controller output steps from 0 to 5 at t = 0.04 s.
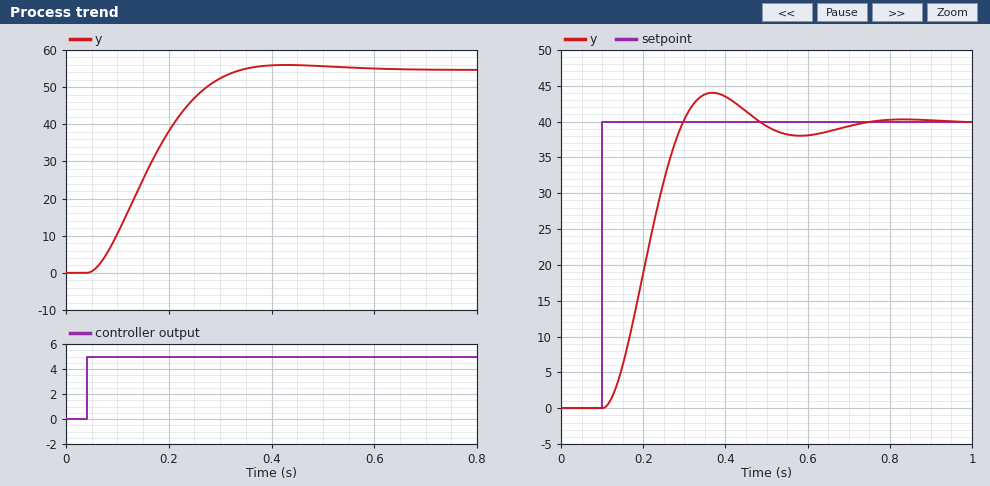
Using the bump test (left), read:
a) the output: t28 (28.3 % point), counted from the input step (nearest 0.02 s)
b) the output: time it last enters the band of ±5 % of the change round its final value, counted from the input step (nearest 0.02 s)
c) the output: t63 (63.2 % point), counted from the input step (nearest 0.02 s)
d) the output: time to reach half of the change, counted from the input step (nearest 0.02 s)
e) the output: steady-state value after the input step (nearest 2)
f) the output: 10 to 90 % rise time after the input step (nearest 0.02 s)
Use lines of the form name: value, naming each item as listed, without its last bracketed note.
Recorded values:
the output: t28 (28.3 % point), counted from the input step: 0.08 s
the output: time it last enters the band of ±5 % of the change round its final value, counted from the input step: 0.26 s
the output: t63 (63.2 % point), counted from the input step: 0.14 s
the output: time to reach half of the change, counted from the input step: 0.12 s
the output: steady-state value after the input step: 54
the output: 10 to 90 % rise time after the input step: 0.18 s
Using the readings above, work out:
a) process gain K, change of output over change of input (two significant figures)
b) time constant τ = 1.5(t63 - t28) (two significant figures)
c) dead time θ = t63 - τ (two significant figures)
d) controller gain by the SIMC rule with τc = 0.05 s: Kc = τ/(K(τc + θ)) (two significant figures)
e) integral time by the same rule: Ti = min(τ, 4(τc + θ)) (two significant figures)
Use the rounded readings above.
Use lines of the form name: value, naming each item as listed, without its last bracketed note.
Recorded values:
process gain K, change of output over change of input: 11
time constant τ = 1.5(t63 - t28): 0.090 s
dead time θ = t63 - τ: 0.050 s
controller gain by the SIMC rule with τc = 0.05 s: Kc = τ/(K(τc + θ)): 0.082
integral time by the same rule: Ti = min(τ, 4(τc + θ)): 0.090 s
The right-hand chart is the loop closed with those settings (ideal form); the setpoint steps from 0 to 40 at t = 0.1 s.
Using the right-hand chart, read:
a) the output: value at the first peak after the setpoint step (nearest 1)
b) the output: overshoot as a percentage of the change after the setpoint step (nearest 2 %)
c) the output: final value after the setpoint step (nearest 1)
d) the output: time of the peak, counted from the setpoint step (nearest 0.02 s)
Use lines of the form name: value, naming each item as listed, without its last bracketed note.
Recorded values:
the output: value at the first peak after the setpoint step: 44
the output: overshoot as a percentage of the change after the setpoint step: 10 %
the output: final value after the setpoint step: 40
the output: time of the peak, counted from the setpoint step: 0.26 s
